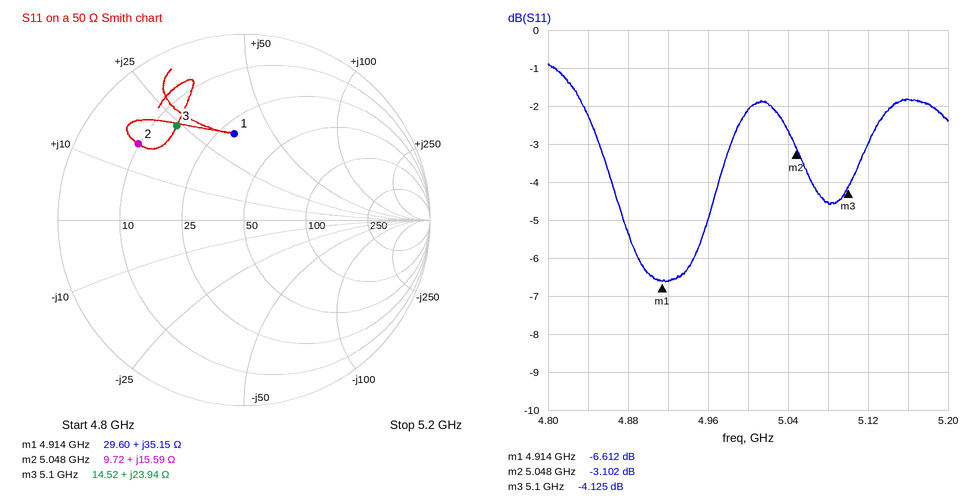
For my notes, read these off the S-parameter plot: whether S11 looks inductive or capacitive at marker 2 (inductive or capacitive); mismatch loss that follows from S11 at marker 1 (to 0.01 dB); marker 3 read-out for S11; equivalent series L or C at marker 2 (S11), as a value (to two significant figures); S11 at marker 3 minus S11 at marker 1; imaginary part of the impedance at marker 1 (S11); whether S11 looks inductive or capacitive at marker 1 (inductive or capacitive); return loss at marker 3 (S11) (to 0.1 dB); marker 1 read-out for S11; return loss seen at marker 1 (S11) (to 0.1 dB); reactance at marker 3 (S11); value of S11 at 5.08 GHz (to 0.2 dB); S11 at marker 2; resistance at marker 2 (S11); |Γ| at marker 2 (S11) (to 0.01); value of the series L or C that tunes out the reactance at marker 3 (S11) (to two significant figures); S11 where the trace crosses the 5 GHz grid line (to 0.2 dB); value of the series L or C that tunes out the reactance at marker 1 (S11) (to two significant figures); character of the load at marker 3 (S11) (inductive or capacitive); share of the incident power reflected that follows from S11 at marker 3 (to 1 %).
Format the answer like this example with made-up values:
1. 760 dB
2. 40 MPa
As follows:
1. inductive
2. 1.07 dB
3. -4.125 dB
4. 490 pH
5. 2.487 dB
6. +35.15 Ω
7. inductive
8. 4.1 dB
9. -6.612 dB
10. 6.6 dB
11. +23.94 Ω
12. -4.6 dB
13. -3.102 dB
14. 9.72 Ω
15. 0.70
16. 1.3 pF
17. -2.0 dB
18. 920 fF
19. inductive
20. 39 %
